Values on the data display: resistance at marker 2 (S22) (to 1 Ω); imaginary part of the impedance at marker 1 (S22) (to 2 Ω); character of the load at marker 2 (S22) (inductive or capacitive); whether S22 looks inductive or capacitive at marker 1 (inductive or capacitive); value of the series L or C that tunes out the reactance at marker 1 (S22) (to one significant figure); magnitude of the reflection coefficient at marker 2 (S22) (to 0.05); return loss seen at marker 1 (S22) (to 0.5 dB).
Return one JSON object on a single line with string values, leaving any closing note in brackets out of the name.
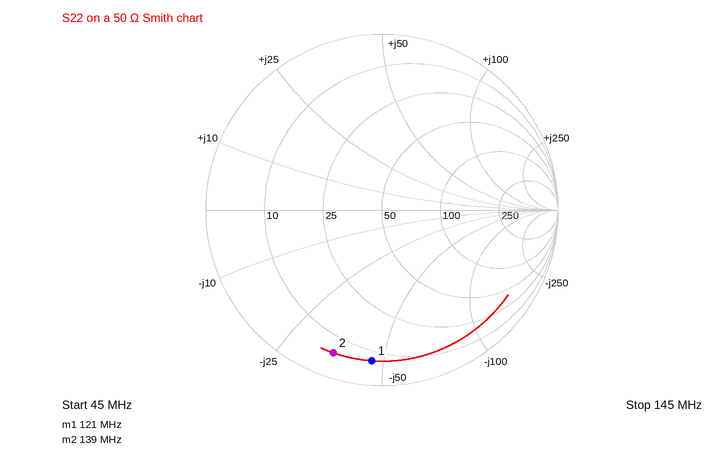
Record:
{"resistance at marker 2 (S22)": "6 Ω", "imaginary part of the impedance at marker 1 (S22)": "-46 Ω", "character of the load at marker 2 (S22)": "capacitive", "whether S22 looks inductive or capacitive at marker 1": "capacitive", "value of the series L or C that tunes out the reactance at marker 1 (S22)": "60 nH", "magnitude of the reflection coefficient at marker 2 (S22)": "0.85", "return loss seen at marker 1 (S22)": "1.5 dB"}
